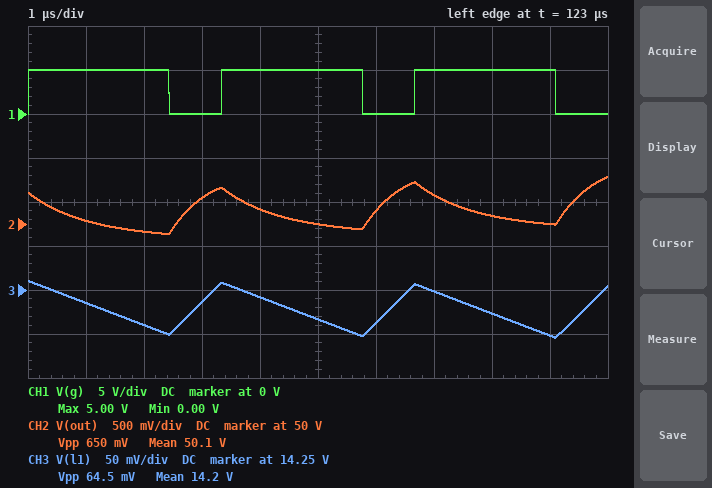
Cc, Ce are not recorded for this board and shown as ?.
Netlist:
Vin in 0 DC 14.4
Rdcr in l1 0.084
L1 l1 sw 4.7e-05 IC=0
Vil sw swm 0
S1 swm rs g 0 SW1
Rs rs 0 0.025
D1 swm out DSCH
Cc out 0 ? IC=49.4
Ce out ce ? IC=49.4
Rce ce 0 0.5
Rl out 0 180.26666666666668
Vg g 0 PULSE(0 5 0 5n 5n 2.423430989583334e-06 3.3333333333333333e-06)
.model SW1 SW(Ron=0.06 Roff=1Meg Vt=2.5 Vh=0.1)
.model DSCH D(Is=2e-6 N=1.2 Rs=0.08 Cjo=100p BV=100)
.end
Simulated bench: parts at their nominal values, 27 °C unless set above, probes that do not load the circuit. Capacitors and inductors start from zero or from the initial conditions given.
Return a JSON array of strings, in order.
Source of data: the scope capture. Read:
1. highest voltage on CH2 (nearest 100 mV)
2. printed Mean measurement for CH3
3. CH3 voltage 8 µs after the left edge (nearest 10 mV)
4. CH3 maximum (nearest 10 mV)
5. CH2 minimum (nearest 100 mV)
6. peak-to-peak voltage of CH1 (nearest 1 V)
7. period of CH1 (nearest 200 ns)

["50.5 V", "14.2 V", "14.22 V", "14.26 V", "49.9 V", "5 V", "3.4 µs"]
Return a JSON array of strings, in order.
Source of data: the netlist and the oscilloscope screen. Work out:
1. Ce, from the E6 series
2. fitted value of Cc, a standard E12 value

["15 µF", "2.2 µF"]
